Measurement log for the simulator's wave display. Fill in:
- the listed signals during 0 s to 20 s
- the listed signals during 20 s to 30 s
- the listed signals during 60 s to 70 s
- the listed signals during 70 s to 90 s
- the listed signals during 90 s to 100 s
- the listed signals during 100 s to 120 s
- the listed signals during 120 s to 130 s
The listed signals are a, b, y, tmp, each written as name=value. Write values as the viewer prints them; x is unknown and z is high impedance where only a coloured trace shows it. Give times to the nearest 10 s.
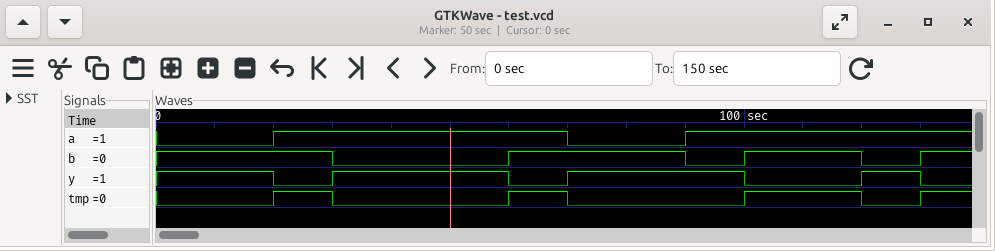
a=0, b=1, y=1, tmp=0
a=1, b=1, y=0, tmp=1
a=1, b=1, y=0, tmp=1
a=0, b=1, y=1, tmp=0
a=1, b=0, y=1, tmp=0
a=1, b=1, y=0, tmp=1
a=1, b=0, y=1, tmp=0
